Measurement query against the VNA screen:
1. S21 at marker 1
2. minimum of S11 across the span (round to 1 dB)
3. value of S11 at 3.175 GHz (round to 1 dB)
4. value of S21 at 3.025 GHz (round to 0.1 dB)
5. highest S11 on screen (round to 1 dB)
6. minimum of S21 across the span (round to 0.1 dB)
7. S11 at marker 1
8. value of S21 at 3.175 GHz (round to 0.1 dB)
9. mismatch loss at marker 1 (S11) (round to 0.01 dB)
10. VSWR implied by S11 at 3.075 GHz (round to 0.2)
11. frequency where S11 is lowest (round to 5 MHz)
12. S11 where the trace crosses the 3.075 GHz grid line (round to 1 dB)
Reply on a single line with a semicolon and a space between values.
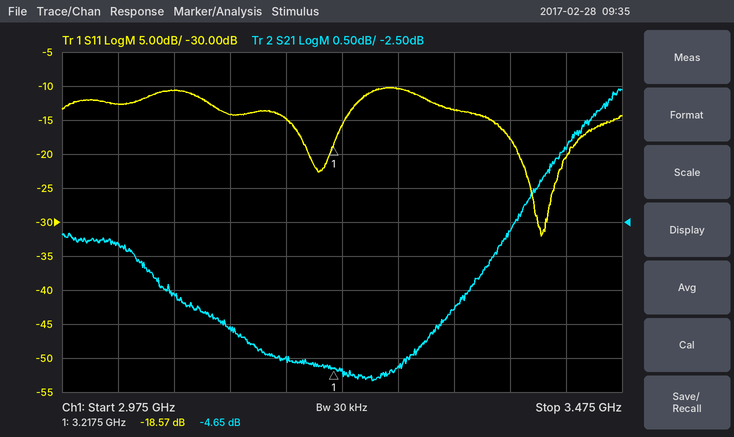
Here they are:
-4.65 dB; -32 dB; -15 dB; -2.8 dB; -10 dB; -4.8 dB; -18.57 dB; -4.5 dB; 0.06 dB; 1.8; 3.405 GHz; -11 dB
